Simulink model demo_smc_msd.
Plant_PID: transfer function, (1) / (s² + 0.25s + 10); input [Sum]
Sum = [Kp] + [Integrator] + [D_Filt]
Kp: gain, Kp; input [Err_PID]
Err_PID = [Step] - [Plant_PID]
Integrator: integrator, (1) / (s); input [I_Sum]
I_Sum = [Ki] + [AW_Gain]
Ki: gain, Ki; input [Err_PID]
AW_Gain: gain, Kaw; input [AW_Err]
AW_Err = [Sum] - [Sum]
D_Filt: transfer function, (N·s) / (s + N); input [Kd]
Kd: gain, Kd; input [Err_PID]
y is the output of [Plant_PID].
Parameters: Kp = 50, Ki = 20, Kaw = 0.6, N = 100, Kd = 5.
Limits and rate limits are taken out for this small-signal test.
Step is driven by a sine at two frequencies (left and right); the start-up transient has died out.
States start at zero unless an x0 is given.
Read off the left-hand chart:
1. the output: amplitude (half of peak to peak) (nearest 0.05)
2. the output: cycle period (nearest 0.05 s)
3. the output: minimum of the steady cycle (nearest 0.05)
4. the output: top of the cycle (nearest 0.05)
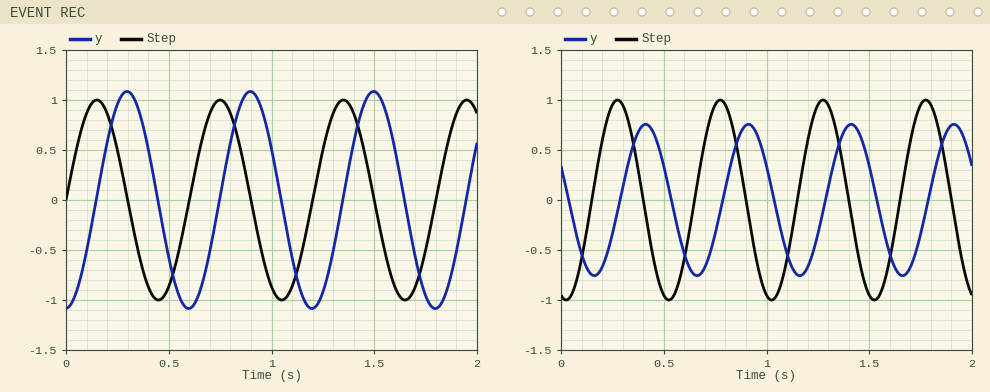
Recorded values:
1.10
0.60 s
-1.10
1.10
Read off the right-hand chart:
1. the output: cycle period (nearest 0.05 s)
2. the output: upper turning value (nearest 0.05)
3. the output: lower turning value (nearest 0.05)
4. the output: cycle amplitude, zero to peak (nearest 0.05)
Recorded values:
0.50 s
0.75
-0.75
0.75
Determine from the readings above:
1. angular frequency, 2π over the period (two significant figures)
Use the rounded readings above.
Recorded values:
13 rad/s
